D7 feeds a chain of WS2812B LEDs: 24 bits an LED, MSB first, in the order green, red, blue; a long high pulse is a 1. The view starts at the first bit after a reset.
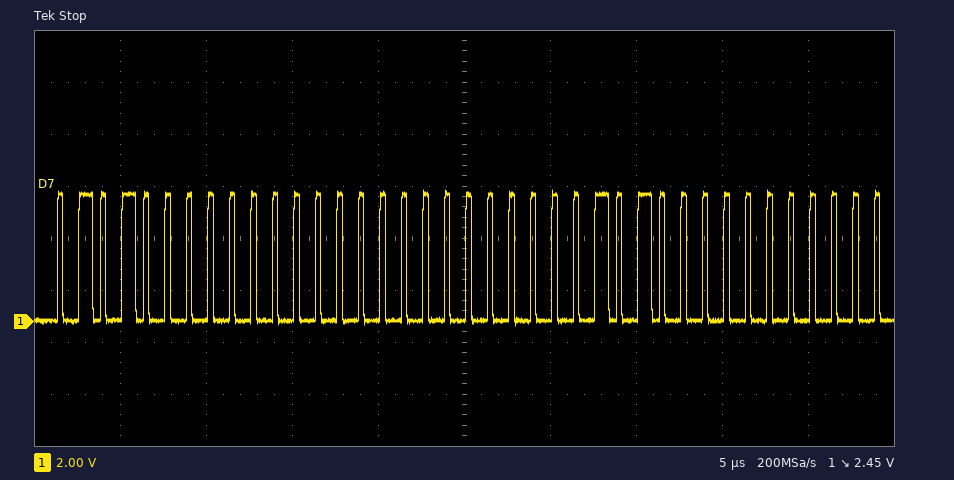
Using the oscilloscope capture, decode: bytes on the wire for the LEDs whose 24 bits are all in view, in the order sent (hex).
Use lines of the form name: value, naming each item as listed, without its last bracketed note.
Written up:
bytes on the wire for the LEDs whose 24 bits are all in view, in the order sent: 50 00 00
